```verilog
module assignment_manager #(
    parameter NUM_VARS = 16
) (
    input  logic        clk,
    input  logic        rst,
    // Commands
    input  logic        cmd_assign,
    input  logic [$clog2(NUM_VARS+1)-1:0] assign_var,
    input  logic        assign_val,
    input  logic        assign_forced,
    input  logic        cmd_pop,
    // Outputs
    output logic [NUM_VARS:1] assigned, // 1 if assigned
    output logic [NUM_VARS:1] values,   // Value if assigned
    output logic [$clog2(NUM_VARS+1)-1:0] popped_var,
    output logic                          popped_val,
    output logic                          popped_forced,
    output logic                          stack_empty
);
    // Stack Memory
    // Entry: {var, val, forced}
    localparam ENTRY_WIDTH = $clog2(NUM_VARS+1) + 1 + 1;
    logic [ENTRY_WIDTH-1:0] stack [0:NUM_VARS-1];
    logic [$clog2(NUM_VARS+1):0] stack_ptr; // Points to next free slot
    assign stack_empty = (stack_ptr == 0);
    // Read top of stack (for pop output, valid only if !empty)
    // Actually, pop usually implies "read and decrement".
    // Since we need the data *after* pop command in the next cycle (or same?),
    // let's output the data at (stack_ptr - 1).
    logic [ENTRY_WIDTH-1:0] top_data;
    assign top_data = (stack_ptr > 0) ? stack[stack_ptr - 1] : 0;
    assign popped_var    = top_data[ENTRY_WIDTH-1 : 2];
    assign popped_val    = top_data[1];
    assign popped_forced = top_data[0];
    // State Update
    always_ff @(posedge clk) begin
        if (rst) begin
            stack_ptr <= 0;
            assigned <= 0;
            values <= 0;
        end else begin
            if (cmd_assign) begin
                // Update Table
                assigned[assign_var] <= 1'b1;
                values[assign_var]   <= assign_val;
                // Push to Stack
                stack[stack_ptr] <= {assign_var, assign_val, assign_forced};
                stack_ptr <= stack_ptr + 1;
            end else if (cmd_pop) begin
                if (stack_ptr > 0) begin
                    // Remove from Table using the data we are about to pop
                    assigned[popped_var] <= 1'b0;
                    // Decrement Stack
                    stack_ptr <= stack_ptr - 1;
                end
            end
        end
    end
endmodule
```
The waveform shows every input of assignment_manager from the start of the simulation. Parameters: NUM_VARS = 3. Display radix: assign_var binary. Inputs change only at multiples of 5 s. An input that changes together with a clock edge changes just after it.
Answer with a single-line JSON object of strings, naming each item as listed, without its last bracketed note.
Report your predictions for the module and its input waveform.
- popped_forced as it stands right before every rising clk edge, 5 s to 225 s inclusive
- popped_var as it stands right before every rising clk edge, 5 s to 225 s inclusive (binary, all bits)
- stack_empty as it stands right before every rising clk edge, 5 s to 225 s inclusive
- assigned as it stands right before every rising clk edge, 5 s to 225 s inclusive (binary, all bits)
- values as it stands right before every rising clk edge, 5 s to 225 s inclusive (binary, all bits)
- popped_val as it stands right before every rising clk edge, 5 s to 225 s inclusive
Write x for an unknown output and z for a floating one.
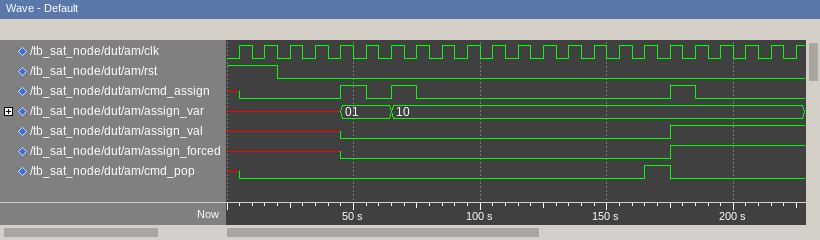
{"popped_forced as it stands right before every rising clk edge, 5 s to 225 s inclusive": "x 0 0 0 0 0 0 0 0 0 0 0 0 0 0 0 0 0 0 1 1 1 1", "popped_var as it stands right before every rising clk edge, 5 s to 225 s inclusive": "x, 00, 00, 00, 00, 00, 01, 01, 10, 10, 10, 10, 10, 10, 10, 10, 10, 10, 01, 10, 10, 10, 10", "stack_empty as it stands right before every rising clk edge, 5 s to 225 s inclusive": "x 1 1 1 1 1 0 0 0 0 0 0 0 0 0 0 0 0 0 0 0 0 0", "assigned as it stands right before every rising clk edge, 5 s to 225 s inclusive": "x, 000, 000, 000, 000, 000, 001, 001, 011, 011, 011, 011, 011, 011, 011, 011, 011, 011, 001, 011, 011, 011, 011", "values as it stands right before every rising clk edge, 5 s to 225 s inclusive": "x, 000, 000, 000, 000, 000, 000, 000, 000, 000, 000, 000, 000, 000, 000, 000, 000, 000, 000, 010, 010, 010, 010", "popped_val as it stands right before every rising clk edge, 5 s to 225 s inclusive": "x 0 0 0 0 0 0 0 0 0 0 0 0 0 0 0 0 0 0 1 1 1 1"}
